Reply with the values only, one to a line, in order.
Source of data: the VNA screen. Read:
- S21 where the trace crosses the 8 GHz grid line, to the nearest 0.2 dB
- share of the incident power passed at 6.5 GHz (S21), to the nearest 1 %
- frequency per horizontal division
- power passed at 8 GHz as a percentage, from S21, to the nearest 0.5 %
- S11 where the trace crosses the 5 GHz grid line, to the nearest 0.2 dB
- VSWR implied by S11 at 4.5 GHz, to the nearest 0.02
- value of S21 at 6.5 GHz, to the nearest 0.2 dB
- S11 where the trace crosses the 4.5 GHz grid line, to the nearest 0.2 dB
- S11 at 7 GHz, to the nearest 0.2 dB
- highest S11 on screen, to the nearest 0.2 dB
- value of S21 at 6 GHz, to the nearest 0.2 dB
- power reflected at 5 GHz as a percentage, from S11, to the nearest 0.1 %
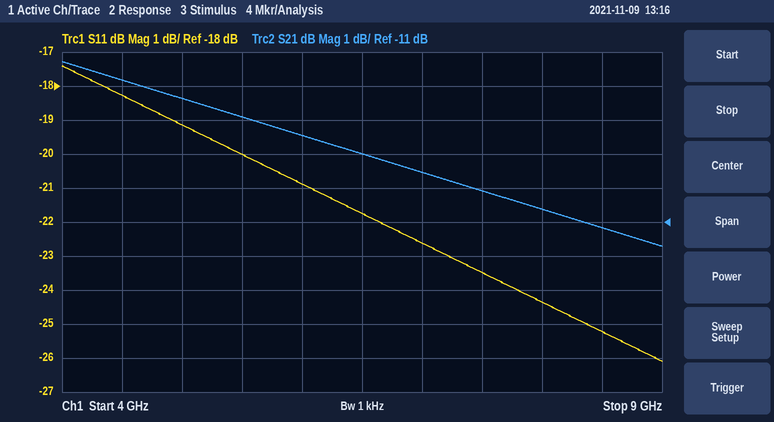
-10.6 dB
13 %
500 MHz
8.5 %
-19.2 dB
1.28
-9.0 dB
-18.2 dB
-22.6 dB
-17.4 dB
-8.4 dB
1.2 %
